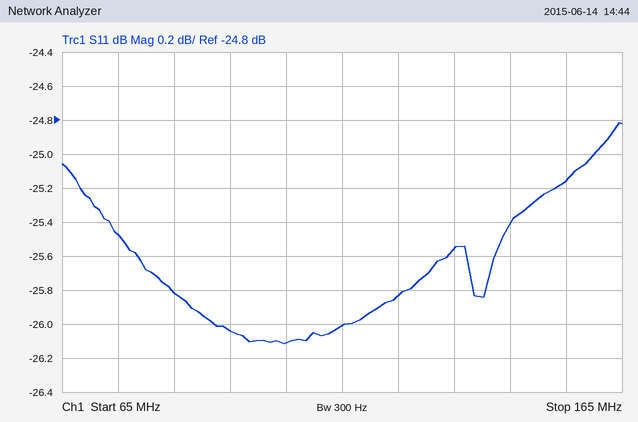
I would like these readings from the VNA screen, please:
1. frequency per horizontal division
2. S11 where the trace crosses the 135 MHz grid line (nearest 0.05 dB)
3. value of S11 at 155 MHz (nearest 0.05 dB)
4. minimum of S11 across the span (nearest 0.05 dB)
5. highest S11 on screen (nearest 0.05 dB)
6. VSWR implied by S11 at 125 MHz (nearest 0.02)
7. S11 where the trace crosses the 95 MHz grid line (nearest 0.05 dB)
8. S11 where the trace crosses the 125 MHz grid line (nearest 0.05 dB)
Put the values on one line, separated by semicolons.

10 MHz; -25.55 dB; -25.15 dB; -26.10 dB; -24.80 dB; 1.10; -26.05 dB; -25.85 dB
